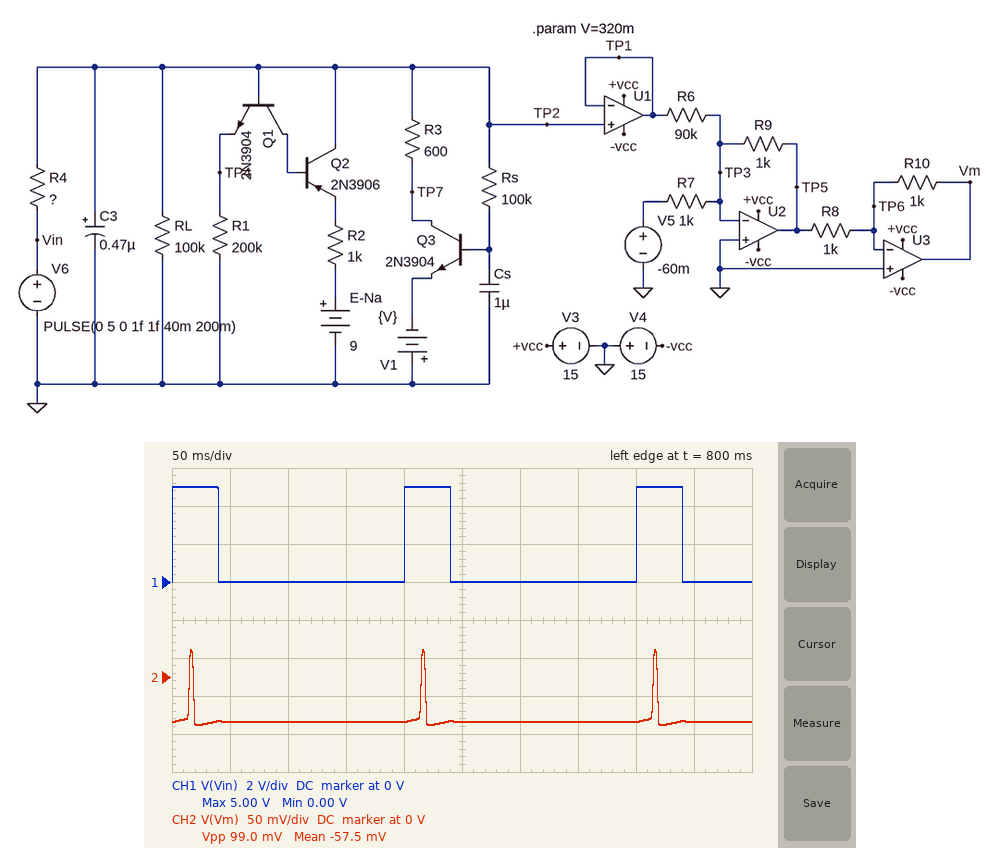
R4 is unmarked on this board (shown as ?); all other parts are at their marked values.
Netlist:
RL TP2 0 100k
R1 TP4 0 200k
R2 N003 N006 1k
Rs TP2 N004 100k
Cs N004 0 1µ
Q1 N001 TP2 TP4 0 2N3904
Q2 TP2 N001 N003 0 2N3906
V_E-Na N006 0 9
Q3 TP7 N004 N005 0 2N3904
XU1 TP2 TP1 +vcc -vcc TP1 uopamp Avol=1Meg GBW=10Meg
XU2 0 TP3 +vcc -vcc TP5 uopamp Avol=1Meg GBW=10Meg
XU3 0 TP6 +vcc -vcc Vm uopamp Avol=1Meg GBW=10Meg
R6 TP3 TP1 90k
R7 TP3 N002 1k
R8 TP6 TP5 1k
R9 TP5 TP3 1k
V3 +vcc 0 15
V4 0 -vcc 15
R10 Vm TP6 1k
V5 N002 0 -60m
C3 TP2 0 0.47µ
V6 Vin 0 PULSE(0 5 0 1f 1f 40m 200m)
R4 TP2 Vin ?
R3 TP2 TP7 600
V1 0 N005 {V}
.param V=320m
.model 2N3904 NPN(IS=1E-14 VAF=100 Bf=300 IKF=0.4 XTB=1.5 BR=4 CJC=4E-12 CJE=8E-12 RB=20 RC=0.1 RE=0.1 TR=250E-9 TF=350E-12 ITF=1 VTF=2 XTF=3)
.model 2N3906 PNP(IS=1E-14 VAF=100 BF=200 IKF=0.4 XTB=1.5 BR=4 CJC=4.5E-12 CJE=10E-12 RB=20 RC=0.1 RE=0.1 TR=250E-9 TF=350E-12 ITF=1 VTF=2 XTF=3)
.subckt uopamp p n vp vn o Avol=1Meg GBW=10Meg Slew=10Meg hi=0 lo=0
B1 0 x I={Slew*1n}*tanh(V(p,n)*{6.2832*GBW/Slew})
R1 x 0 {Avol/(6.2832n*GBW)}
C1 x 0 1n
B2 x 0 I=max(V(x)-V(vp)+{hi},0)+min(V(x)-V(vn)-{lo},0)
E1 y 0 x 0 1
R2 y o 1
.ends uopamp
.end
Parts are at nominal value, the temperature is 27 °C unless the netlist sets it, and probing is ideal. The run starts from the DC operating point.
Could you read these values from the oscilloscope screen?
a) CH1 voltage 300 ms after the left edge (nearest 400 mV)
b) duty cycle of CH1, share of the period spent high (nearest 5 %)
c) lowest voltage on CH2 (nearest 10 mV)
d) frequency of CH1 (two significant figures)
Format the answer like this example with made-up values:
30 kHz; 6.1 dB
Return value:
0 V; 20 %; -60 mV; 5.0 Hz
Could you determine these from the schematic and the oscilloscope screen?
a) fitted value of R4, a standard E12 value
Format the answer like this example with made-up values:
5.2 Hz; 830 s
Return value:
270 kΩ
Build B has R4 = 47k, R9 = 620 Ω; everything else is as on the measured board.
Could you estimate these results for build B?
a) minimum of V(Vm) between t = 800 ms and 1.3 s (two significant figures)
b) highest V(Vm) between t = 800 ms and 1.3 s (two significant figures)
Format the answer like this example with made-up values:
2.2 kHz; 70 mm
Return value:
-39 mV; 22 mV
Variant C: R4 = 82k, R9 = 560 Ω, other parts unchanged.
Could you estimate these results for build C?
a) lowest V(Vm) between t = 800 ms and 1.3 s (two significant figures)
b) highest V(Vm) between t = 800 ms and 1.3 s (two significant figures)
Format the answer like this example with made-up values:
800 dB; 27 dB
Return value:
-35 mV; 20 mV
